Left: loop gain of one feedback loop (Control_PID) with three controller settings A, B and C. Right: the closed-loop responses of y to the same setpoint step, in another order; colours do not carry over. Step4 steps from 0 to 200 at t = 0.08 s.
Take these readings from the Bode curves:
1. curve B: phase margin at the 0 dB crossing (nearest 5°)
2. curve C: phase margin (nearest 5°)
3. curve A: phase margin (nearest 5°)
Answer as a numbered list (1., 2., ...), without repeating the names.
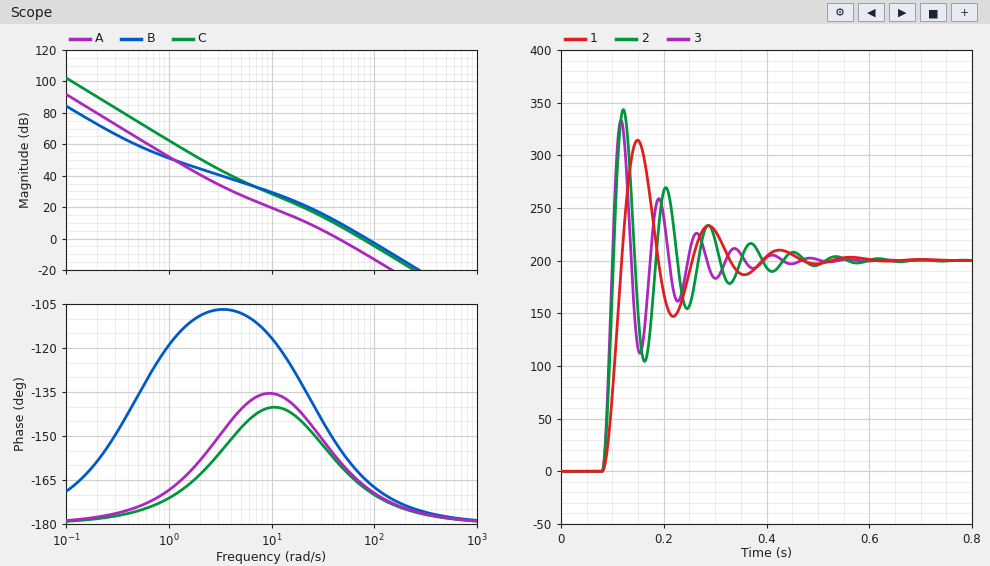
1. 15°
2. 15°
3. 20°
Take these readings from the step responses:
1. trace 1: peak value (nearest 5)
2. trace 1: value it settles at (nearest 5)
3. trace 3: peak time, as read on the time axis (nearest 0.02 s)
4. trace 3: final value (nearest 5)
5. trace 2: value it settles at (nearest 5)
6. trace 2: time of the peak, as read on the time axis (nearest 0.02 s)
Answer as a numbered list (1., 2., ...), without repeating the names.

1. 315
2. 200
3. 0.12 s
4. 200
5. 200
6. 0.12 s
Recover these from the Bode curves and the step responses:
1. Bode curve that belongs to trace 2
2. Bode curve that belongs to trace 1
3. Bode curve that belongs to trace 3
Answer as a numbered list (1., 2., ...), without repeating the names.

1. C
2. A
3. B
